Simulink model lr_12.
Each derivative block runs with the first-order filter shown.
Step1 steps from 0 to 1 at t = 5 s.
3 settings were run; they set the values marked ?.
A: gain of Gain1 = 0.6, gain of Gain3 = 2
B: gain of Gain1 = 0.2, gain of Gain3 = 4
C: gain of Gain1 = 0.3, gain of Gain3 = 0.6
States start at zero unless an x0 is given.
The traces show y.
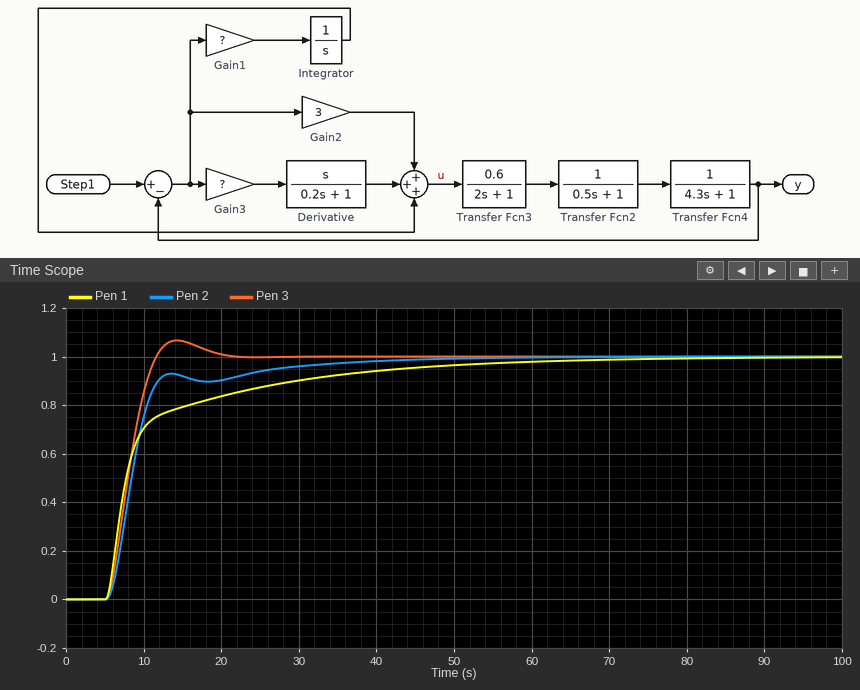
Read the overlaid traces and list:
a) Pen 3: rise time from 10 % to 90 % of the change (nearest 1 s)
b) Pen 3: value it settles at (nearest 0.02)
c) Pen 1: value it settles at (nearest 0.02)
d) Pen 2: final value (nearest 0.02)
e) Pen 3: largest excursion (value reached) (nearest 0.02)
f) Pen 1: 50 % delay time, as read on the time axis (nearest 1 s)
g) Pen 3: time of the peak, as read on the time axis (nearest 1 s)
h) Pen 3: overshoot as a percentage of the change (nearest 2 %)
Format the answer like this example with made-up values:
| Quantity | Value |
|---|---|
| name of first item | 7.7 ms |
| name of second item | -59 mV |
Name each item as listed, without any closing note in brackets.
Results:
| Quantity | Value |
|---|---|
| Pen 3: rise time from 10 % to 90 % of the change | 4 s |
| Pen 3: value it settles at | 1.00 |
| Pen 1: value it settles at | 1.00 |
| Pen 2: final value | 1.00 |
| Pen 3: largest excursion (value reached) | 1.06 |
| Pen 1: 50 % delay time, as read on the time axis | 8 s |
| Pen 3: time of the peak, as read on the time axis | 14 s |
| Pen 3: overshoot as a percentage of the change | 6 % |
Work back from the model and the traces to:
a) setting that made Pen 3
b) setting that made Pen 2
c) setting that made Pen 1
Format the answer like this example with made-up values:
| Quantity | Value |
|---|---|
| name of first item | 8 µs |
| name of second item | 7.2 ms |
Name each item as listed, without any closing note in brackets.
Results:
| Quantity | Value |
|---|---|
| setting that made Pen 3 | A |
| setting that made Pen 2 | C |
| setting that made Pen 1 | B |
